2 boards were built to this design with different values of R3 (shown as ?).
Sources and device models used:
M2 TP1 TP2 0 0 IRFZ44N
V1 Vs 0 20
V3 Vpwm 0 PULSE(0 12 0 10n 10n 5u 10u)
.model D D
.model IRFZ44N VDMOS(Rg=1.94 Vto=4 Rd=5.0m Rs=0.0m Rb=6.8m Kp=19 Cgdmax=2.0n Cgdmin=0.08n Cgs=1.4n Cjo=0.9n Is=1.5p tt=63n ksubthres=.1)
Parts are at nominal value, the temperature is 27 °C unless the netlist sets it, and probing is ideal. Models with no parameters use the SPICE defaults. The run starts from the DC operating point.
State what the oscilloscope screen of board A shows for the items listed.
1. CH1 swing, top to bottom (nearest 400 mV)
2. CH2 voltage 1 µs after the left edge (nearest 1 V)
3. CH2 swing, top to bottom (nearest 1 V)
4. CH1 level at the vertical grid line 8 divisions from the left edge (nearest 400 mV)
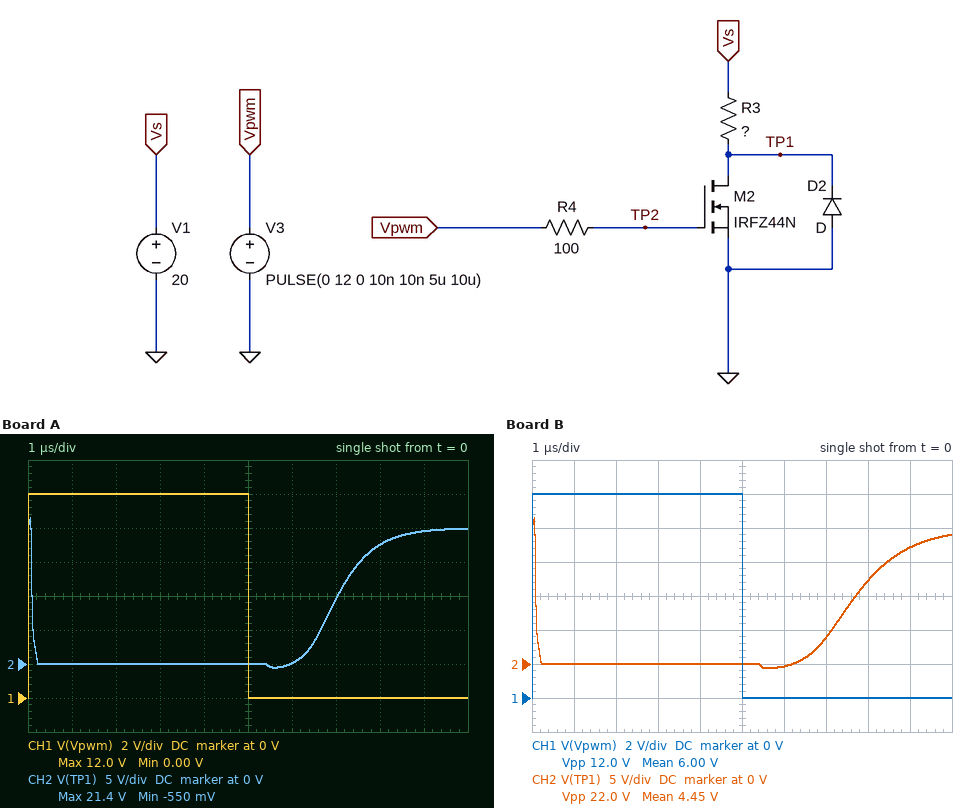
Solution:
12.0 V
0 V
22 V
0 V
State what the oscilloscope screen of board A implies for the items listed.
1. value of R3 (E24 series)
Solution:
2 kΩ
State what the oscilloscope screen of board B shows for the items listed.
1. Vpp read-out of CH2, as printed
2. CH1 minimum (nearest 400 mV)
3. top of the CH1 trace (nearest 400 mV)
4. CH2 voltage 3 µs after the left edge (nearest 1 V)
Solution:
22.0 V
0 V
12.0 V
0 V
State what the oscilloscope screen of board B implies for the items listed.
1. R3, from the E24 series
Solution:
3 kΩ
